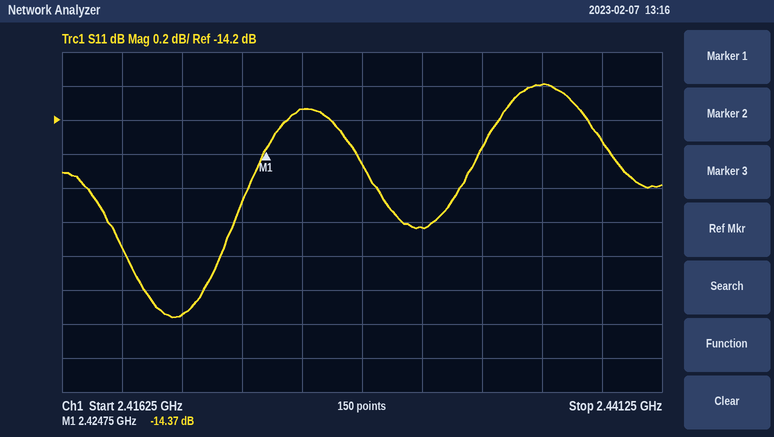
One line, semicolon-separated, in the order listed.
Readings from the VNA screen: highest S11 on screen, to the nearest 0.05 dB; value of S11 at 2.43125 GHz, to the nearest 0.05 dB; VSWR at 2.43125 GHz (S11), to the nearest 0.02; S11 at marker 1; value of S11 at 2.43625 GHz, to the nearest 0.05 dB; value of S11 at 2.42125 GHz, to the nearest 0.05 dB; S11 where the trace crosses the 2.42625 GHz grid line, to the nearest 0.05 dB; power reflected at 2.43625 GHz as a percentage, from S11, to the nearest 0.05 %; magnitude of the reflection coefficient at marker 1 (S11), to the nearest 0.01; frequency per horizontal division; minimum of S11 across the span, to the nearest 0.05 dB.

-14.00 dB; -14.85 dB; 1.44; -14.37 dB; -14.00 dB; -15.35 dB; -14.15 dB; 4.00 %; 0.19; 2.5 MHz; -15.35 dB
